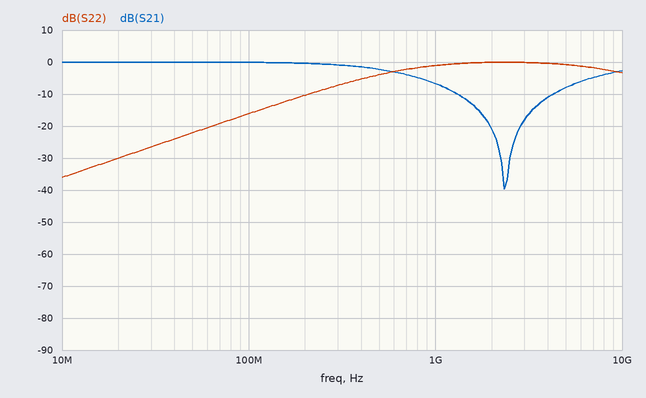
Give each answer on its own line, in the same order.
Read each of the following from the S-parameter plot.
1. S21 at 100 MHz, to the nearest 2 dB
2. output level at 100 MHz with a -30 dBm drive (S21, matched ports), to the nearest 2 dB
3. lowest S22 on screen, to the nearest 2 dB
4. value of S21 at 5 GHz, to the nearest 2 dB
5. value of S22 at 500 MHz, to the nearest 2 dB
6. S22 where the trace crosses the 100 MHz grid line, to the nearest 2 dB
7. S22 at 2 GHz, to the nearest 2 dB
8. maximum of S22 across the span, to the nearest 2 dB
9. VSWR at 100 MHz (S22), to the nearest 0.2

0 dB
-30 dBm
-36 dB
-8 dB
-4 dB
-16 dB
0 dB
0 dB
1.4
